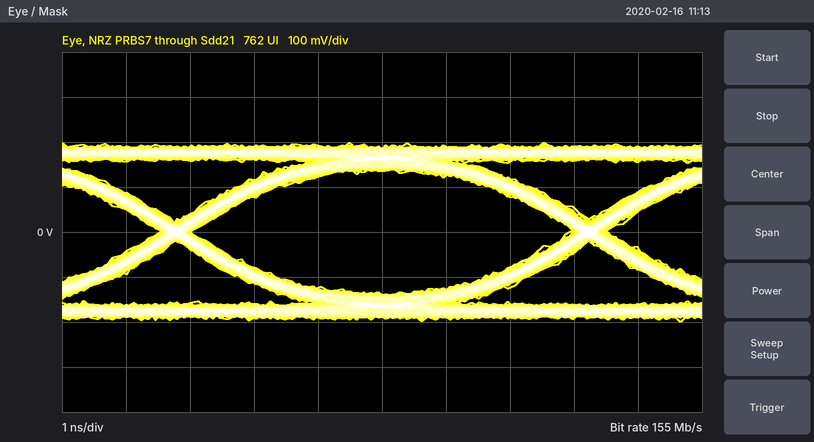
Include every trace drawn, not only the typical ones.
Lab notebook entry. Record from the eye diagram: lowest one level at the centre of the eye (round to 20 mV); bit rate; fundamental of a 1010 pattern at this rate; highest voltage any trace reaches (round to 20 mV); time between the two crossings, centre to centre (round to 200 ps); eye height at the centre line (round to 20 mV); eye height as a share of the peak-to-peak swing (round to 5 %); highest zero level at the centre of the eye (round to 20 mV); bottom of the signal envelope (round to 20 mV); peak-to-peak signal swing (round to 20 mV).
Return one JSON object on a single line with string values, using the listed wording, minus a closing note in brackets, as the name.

{"lowest one level at the centre of the eye": "140 mV", "bit rate": "155 Mb/s", "fundamental of a 1010 pattern at this rate": "77.5 MHz", "highest voltage any trace reaches": "200 mV", "time between the two crossings, centre to centre": "6.4 ns", "eye height at the centre line": "280 mV", "eye height as a share of the peak-to-peak swing": "70 %", "highest zero level at the centre of the eye": "-140 mV", "bottom of the signal envelope": "-200 mV", "peak-to-peak signal swing": "400 mV"}
